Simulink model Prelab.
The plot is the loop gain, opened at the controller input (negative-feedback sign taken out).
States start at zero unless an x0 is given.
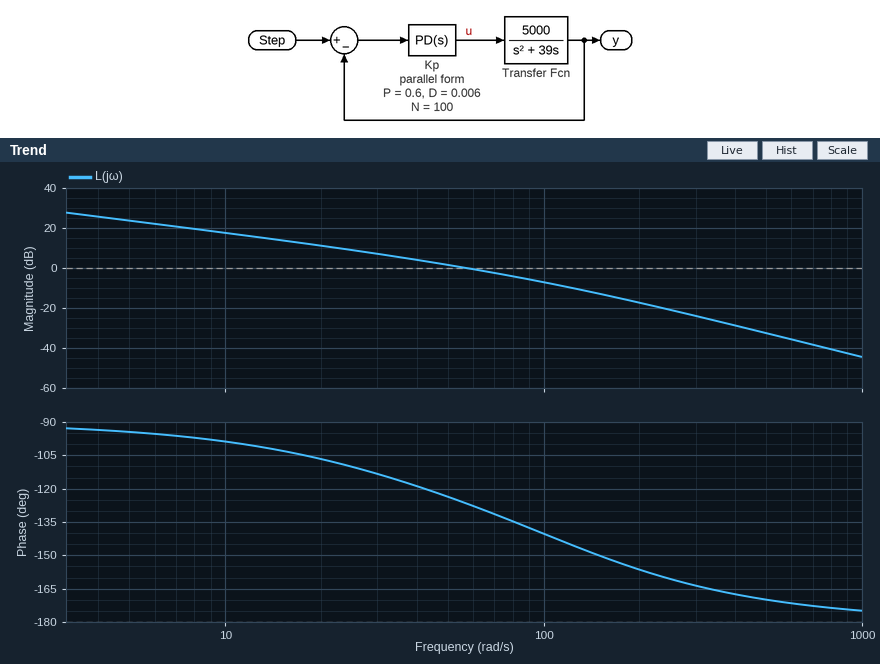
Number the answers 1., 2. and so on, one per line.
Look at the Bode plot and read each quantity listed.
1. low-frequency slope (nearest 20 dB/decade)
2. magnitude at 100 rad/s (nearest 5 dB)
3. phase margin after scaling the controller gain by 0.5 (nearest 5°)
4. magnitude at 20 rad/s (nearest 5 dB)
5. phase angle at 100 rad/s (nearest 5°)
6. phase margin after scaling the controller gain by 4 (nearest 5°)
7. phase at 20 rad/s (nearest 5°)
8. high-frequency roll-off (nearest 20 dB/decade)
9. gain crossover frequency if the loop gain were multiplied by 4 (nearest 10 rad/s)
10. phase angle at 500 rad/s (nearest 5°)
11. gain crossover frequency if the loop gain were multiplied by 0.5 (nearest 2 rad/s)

1. -20 dB/decade
2. -5 dB
3. 65°
4. 10 dB
5. -140°
6. 30°
7. -105°
8. -40 dB/decade
9. 140 rad/s
10. -170°
11. 34 rad/s
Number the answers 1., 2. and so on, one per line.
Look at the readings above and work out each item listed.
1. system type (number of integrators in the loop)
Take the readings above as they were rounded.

1. 1
